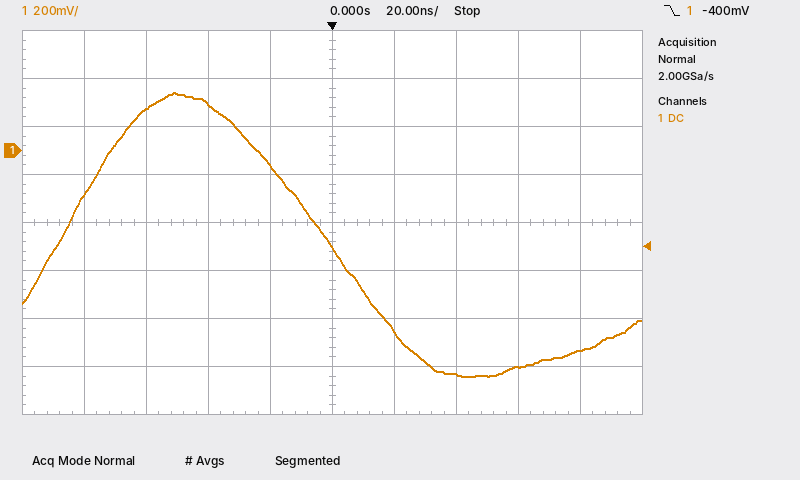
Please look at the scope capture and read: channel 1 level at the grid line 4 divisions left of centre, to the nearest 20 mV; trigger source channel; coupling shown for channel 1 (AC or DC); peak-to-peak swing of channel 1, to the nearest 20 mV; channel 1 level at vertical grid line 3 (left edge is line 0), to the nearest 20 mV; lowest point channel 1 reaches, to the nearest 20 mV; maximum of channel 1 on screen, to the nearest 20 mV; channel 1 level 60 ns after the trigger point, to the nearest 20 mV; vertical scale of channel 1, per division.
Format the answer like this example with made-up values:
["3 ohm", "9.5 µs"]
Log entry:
["-180 mV", "channel 1", "DC", "1.18 V", "200 mV", "-940 mV", "240 mV", "-900 mV", "200 mV"]
